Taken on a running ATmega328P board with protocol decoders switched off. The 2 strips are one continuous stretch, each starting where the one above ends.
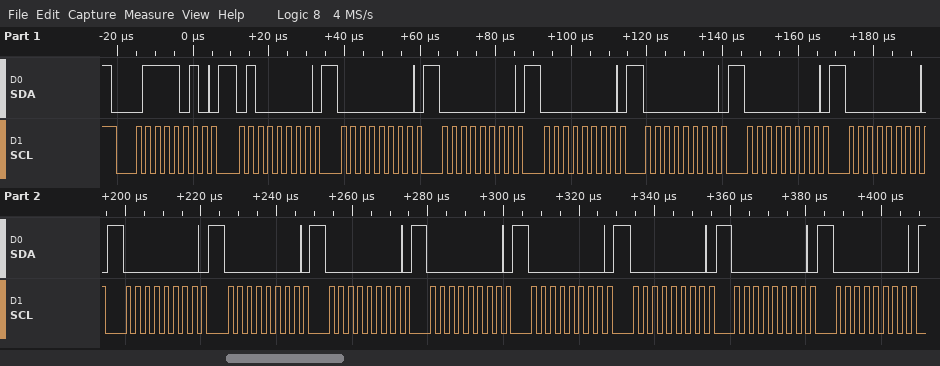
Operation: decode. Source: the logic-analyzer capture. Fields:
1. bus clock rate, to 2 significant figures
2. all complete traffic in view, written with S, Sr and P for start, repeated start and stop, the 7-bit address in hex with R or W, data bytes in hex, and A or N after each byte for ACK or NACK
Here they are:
400 kHz
S 3DW A 40 A 00 A 00 A 00 A 00 A 00 A 00 A 00 A 00 A 00 A 00 A 00 A 00 A 00 A 00 A
